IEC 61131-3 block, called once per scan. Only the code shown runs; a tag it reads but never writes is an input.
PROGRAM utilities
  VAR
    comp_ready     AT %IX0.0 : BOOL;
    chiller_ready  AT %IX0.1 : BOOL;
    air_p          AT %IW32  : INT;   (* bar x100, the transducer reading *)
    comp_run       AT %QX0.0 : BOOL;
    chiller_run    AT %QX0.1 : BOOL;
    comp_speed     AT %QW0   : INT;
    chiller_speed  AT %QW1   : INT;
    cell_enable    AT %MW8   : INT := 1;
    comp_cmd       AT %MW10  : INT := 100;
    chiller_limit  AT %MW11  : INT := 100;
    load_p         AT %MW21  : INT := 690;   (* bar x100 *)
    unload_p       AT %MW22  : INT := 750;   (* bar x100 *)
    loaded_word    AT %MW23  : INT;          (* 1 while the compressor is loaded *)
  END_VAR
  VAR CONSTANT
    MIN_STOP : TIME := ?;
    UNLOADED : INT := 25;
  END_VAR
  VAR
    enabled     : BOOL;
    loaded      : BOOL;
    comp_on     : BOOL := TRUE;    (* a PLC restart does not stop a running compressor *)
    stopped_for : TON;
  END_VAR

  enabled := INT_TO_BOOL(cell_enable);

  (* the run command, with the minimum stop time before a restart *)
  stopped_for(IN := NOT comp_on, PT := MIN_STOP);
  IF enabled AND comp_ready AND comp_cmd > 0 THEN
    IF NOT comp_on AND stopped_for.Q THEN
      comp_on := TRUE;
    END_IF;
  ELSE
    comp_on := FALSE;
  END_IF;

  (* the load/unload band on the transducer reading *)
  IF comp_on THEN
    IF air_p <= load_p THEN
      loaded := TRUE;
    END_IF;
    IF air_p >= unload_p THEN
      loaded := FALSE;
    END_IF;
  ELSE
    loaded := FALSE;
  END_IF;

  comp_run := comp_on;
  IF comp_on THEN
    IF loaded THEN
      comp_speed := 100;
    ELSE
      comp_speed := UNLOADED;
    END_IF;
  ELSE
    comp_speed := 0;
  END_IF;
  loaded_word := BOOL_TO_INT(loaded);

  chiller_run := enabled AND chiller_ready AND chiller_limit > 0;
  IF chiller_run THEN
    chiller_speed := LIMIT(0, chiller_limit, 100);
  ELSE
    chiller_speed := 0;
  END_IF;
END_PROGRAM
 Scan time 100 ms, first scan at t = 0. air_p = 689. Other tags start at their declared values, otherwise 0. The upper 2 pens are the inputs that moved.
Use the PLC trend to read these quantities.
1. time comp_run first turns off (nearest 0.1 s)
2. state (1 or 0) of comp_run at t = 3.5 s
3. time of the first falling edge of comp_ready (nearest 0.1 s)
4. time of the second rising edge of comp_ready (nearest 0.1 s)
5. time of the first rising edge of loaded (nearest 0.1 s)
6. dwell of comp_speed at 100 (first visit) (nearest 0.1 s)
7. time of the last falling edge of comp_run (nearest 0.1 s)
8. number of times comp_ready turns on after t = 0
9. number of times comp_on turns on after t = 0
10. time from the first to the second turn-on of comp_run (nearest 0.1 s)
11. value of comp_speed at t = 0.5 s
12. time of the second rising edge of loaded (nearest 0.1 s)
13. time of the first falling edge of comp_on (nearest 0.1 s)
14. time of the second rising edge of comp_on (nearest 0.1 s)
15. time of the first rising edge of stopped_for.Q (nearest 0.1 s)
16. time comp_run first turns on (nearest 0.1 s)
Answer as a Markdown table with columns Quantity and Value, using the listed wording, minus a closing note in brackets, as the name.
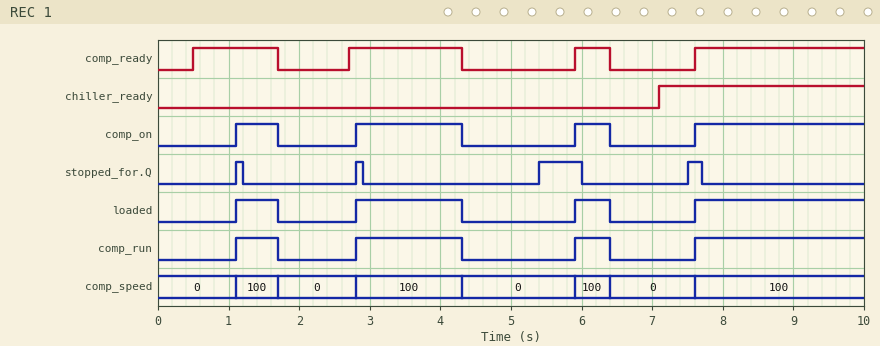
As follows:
| Quantity | Value |
|---|---|
| time comp_run first turns off | 1.7 s |
| state (1 or 0) of comp_run at t = 3.5 s | 1 |
| time of the first falling edge of comp_ready | 1.7 s |
| time of the second rising edge of comp_ready | 2.7 s |
| time of the first rising edge of loaded | 1.1 s |
| dwell of comp_speed at 100 (first visit) | 0.6 s |
| time of the last falling edge of comp_run | 6.4 s |
| number of times comp_ready turns on after t = 0 | 4 |
| number of times comp_on turns on after t = 0 | 4 |
| time from the first to the second turn-on of comp_run | 1.7 s |
| value of comp_speed at t = 0.5 s | 0 |
| time of the second rising edge of loaded | 2.8 s |
| time of the first falling edge of comp_on | 1.7 s |
| time of the second rising edge of comp_on | 2.8 s |
| time of the first rising edge of stopped_for.Q | 1.1 s |
| time comp_run first turns on | 1.1 s |
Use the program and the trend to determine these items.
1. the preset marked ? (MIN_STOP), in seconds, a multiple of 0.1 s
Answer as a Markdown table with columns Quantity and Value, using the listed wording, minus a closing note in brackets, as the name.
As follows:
| Quantity | Value |
|---|---|
| the preset marked ? (MIN_STOP), in seconds, a multiple of 0.1 s | 1.0 s |
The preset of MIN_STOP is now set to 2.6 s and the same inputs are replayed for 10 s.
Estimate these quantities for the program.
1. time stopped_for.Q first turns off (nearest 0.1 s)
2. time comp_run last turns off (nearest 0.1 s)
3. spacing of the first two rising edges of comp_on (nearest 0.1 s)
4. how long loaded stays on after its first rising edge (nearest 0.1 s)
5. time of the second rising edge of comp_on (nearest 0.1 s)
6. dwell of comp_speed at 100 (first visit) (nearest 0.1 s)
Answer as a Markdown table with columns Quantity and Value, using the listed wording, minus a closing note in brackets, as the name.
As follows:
| Quantity | Value |
|---|---|
| time stopped_for.Q first turns off | 2.8 s |
| time comp_run last turns off | 4.3 s |
| spacing of the first two rising edges of comp_on | 4.9 s |
| how long loaded stays on after its first rising edge | 1.6 s |
| time of the second rising edge of comp_on | 7.6 s |
| dwell of comp_speed at 100 (first visit) | 1.6 s |
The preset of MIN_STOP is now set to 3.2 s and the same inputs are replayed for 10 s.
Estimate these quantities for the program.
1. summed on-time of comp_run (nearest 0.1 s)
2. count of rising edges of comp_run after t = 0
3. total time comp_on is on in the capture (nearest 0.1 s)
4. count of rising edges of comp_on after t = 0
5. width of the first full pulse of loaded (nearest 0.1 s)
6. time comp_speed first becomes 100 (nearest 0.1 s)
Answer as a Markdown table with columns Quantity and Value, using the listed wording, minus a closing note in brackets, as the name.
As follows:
| Quantity | Value |
|---|---|
| summed on-time of comp_run | 3.4 s |
| count of rising edges of comp_run after t = 0 | 2 |
| total time comp_on is on in the capture | 3.4 s |
| count of rising edges of comp_on after t = 0 | 2 |
| width of the first full pulse of loaded | 1.0 s |
| time comp_speed first becomes 100 | 3.3 s |
